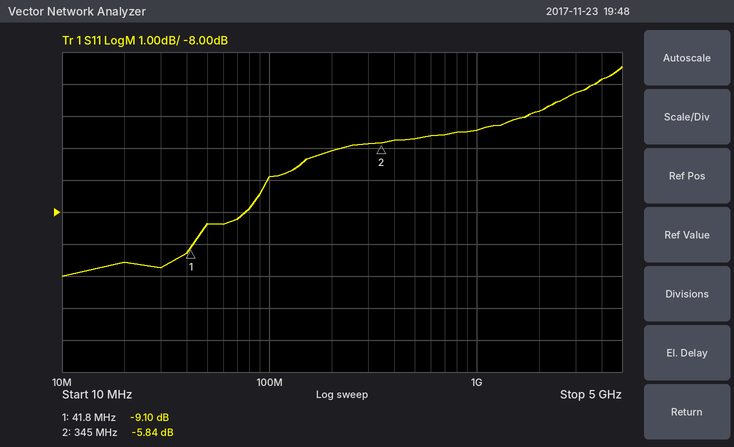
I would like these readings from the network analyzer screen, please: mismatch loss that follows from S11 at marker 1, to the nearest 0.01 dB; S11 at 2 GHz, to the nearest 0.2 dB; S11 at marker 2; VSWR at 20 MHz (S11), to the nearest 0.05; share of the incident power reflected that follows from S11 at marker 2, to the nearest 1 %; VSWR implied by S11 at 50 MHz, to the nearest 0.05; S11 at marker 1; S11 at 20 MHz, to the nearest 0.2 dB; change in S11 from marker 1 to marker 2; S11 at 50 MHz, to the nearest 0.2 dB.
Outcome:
0.57 dB
-4.8 dB
-5.84 dB
2.00
26 %
2.25
-9.10 dB
-9.6 dB
3.26 dB
-8.4 dB
